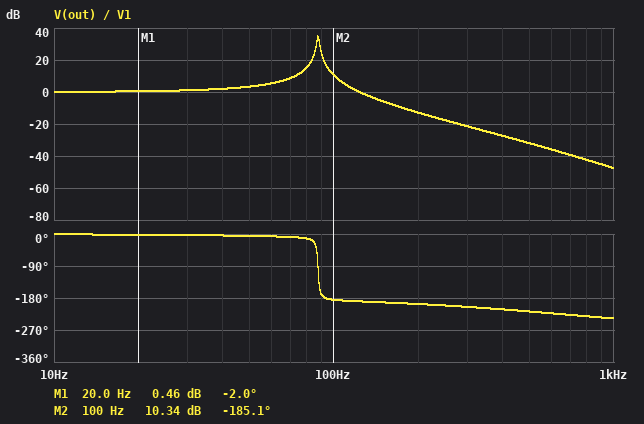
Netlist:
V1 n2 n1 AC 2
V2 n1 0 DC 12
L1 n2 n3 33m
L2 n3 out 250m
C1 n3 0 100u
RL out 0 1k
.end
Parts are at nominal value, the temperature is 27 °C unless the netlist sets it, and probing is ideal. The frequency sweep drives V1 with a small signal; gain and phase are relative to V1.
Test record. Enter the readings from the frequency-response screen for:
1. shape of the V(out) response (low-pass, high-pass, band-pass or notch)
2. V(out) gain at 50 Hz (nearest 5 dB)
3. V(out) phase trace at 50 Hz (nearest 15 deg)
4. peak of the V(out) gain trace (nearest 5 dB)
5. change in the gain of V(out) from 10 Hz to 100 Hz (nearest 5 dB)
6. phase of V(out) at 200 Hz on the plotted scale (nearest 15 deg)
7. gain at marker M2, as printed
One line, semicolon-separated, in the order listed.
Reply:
low-pass; 5 dB; 0 deg; 35 dB; 10 dB; -195 deg; 10.34 dB
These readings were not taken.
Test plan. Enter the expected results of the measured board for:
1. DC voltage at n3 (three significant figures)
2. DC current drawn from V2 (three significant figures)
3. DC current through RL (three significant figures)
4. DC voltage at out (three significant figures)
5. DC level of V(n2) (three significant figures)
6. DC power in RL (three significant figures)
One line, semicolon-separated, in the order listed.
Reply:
12.0 V; 12.0 mA; 12.0 mA; 12.0 V; 12.0 V; 144 mW
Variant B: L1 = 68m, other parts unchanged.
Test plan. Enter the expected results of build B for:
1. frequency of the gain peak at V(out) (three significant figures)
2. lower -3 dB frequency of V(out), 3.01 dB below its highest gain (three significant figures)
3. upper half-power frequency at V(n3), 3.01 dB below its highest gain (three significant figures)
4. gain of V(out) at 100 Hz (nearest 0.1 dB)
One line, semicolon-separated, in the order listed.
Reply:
61.1 Hz; 60.3 Hz; 61.9 Hz; -4.6 dB
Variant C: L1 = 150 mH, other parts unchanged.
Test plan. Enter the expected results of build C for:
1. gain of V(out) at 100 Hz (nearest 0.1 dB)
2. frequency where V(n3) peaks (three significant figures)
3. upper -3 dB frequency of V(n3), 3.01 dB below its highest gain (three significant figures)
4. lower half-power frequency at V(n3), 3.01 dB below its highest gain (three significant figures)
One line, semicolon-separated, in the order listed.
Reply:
-13.9 dB; 41.1 Hz; 41.9 Hz; 40.3 Hz
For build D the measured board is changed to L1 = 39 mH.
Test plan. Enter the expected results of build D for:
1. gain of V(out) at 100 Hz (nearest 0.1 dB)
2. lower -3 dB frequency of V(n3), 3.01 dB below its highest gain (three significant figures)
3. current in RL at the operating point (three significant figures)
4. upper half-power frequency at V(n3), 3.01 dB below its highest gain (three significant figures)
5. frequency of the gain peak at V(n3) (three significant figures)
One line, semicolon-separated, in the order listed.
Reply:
5.3 dB; 79.9 Hz; 12.0 mA; 81.5 Hz; 80.7 Hz
